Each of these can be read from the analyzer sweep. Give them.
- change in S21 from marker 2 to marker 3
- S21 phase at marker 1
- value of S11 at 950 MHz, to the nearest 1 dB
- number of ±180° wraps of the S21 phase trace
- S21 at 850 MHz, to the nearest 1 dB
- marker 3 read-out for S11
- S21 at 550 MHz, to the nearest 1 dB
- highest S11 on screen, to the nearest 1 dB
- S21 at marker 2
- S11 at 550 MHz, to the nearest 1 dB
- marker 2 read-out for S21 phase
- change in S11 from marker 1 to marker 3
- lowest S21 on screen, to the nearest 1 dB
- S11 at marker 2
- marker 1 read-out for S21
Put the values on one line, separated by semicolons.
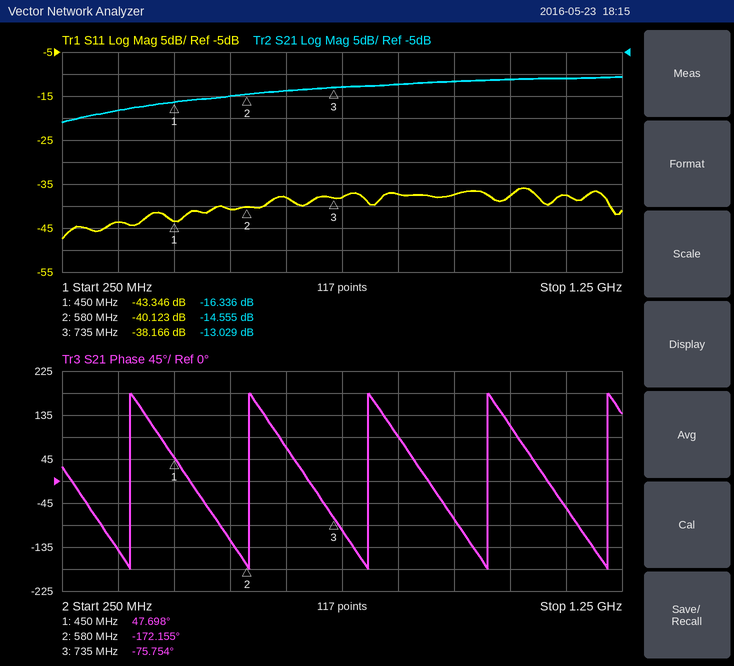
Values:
1.526 dB; 47.698°; -37 dB; 5; -12 dB; -38.166 dB; -15 dB; -36 dB; -14.555 dB; -41 dB; -172.155°; 5.180 dB; -21 dB; -40.123 dB; -16.336 dB
